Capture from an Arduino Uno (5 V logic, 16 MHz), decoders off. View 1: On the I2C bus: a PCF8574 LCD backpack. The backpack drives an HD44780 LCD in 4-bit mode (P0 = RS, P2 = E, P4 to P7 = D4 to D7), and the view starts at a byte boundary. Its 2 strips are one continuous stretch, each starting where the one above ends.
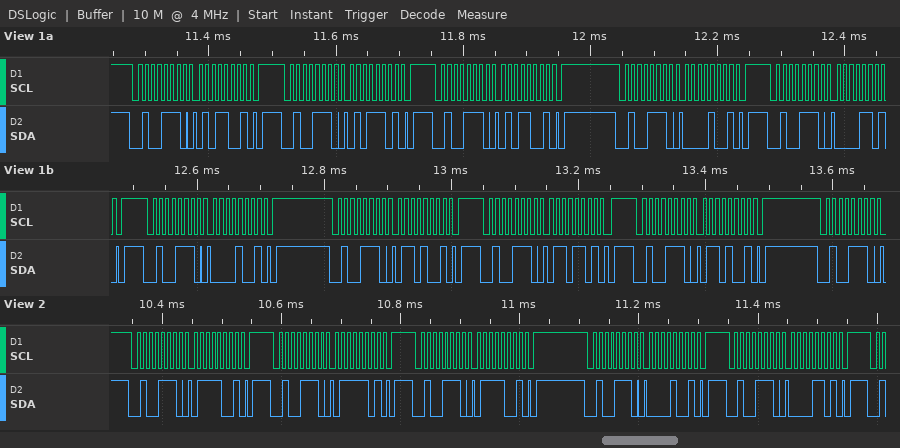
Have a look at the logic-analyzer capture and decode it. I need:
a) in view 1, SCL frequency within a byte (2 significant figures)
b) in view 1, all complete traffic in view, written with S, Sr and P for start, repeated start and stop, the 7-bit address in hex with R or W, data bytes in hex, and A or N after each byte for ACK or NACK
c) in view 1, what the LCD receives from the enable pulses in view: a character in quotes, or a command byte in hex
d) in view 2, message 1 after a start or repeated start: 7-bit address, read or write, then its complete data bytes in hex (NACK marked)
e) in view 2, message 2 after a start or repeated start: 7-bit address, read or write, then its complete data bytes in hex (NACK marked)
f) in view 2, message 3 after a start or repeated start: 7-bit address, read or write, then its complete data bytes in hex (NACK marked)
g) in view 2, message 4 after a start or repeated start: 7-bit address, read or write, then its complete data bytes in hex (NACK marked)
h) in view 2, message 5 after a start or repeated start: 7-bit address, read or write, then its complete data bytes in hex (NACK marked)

100 kHz
S 27W A 59 A P S 27W A 5D A P S 27W A 59 A P S 27W A 09 A P S 27W A 0D A P S 27W A 09 A P S 27W A 69 A P S 27W A 6D A P S 27W A 69 A P S 27W A
'P'
0x27 write: 79
0x27 write: 7D
0x27 write: 79
0x27 write: 09
0x27 write: 0D
